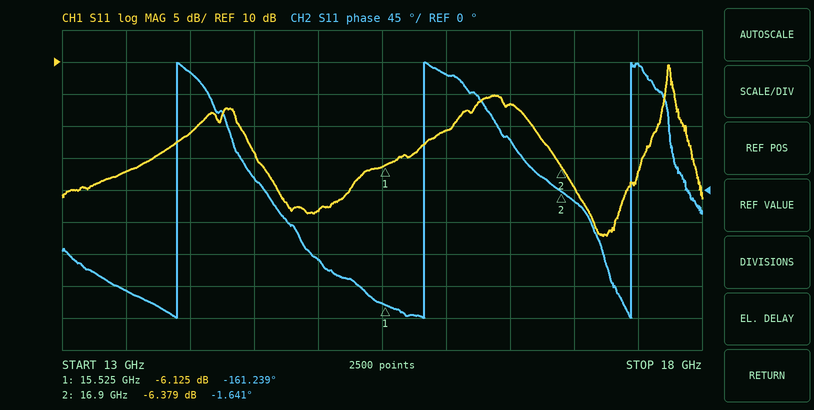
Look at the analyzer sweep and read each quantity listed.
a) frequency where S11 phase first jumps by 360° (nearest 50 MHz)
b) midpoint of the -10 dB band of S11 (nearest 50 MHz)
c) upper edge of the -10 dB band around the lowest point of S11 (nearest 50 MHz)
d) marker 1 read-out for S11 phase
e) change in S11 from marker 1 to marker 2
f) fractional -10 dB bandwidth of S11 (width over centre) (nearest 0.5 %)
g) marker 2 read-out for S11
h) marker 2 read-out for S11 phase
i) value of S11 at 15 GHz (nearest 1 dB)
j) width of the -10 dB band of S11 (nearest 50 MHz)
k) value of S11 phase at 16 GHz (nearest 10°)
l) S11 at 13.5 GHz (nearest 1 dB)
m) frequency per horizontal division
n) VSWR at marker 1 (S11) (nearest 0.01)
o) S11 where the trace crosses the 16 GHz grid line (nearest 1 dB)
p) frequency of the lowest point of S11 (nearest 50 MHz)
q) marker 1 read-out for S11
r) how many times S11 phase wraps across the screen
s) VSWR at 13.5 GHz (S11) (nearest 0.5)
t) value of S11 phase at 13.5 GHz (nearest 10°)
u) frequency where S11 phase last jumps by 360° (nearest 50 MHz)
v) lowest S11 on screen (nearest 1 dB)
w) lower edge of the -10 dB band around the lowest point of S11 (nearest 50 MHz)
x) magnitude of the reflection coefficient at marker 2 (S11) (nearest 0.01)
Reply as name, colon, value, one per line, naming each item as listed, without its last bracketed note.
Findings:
frequency where S11 phase first jumps by 360°: 13.90 GHz
midpoint of the -10 dB band of S11: 17.20 GHz
upper edge of the -10 dB band around the lowest point of S11: 17.40 GHz
marker 1 read-out for S11 phase: -161.239°
change in S11 from marker 1 to marker 2: -0.254 dB
fractional -10 dB bandwidth of S11 (width over centre): 2.5 %
marker 2 read-out for S11: -6.379 dB
marker 2 read-out for S11 phase: -1.641°
value of S11 at 15 GHz: -13 dB
width of the -10 dB band of S11: 400 MHz
value of S11 phase at 16 GHz: 160°
S11 at 13.5 GHz: -7 dB
frequency per horizontal division: 500 MHz
VSWR at marker 1 (S11): 2.95
S11 where the trace crosses the 16 GHz grid line: -1 dB
frequency of the lowest point of S11: 17.25 GHz
marker 1 read-out for S11: -6.125 dB
how many times S11 phase wraps across the screen: 3
VSWR at 13.5 GHz (S11): 2.5
value of S11 phase at 13.5 GHz: -140°
frequency where S11 phase last jumps by 360°: 17.45 GHz
lowest S11 on screen: -17 dB
lower edge of the -10 dB band around the lowest point of S11: 17.00 GHz
magnitude of the reflection coefficient at marker 2 (S11): 0.48
